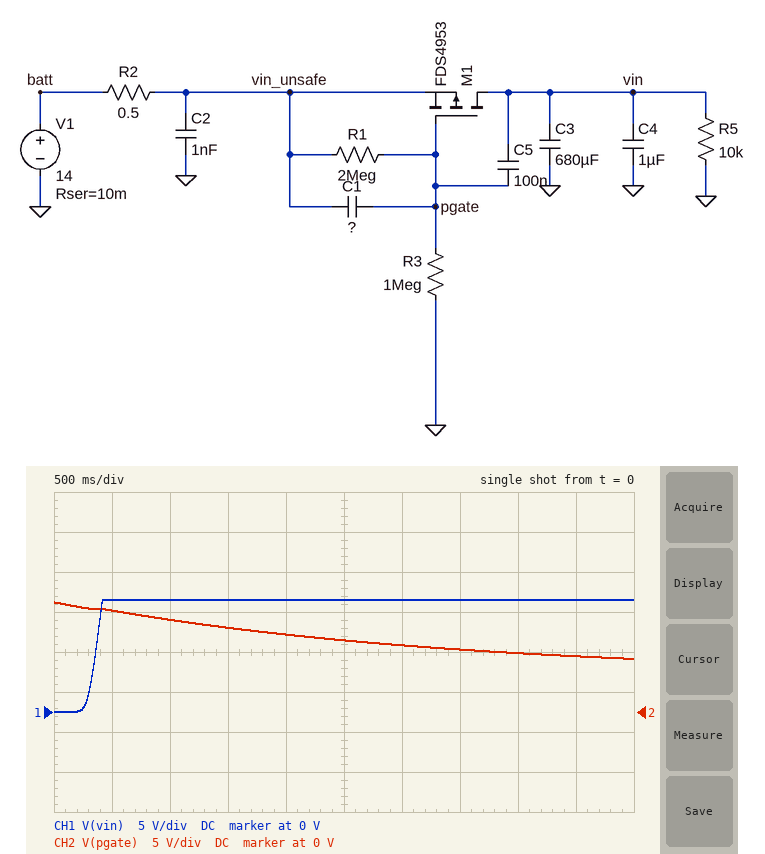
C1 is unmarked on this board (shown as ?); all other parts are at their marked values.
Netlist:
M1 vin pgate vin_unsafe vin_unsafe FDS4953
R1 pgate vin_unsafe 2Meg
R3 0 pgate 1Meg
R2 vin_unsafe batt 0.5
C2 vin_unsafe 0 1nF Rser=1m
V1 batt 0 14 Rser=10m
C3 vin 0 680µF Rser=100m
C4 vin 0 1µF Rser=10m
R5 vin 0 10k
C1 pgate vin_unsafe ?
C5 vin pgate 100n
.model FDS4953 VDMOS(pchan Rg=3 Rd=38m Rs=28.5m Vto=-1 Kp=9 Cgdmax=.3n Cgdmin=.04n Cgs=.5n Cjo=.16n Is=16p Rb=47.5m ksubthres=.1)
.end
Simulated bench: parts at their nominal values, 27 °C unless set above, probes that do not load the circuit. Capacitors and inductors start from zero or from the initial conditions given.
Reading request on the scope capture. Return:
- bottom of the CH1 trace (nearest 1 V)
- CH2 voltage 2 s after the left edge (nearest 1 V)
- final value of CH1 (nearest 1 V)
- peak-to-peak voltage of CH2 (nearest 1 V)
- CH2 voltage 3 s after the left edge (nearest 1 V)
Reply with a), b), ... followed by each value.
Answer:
a) 0 V
b) 10 V
c) 14 V
d) 7 V
e) 8 V
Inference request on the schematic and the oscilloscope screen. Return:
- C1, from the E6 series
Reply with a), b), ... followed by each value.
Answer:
a) 4.7 µF
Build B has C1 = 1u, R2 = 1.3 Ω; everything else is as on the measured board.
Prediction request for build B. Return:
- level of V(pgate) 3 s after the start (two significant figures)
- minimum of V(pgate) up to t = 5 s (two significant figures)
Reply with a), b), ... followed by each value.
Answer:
a) 4.8 V
b) 4.7 V
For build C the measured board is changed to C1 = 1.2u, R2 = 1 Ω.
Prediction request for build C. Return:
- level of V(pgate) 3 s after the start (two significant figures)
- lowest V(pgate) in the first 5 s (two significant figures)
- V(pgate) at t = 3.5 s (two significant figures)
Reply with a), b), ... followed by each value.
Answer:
a) 5.0 V
b) 4.7 V
c) 4.8 V
